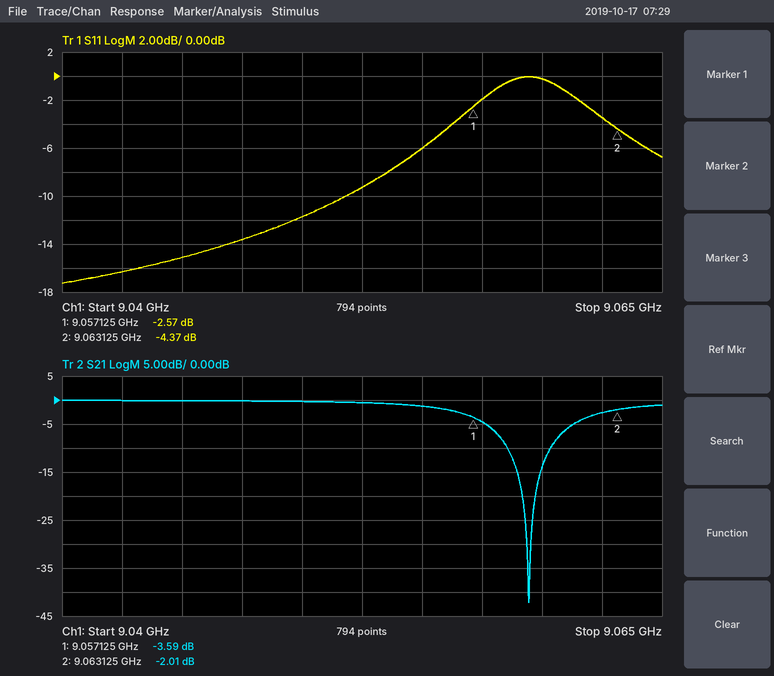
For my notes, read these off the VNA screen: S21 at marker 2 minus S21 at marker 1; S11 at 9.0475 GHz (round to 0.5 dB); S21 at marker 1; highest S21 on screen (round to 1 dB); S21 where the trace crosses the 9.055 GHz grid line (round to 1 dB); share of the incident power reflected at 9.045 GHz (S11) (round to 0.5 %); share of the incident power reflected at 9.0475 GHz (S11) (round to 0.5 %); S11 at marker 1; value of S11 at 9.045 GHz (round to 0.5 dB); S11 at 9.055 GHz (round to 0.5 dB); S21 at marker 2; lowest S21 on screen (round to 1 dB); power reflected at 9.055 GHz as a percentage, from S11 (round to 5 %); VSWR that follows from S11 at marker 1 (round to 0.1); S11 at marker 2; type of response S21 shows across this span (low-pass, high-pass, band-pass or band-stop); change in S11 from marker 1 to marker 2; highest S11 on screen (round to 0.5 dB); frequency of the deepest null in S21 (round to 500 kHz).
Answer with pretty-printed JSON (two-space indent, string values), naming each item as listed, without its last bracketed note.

{
  "S21 at marker 2 minus S21 at marker 1": "1.58 dB",
  "S11 at 9.0475 GHz": "-13.5 dB",
  "S21 at marker 1": "-3.59 dB",
  "highest S21 on screen": "0 dB",
  "S21 where the trace crosses the 9.055 GHz grid line": "-1 dB",
  "share of the incident power reflected at 9.045 GHz (S11)": "3.0 %",
  "share of the incident power reflected at 9.0475 GHz (S11)": "4.5 %",
  "S11 at marker 1": "-2.57 dB",
  "value of S11 at 9.045 GHz": "-15.0 dB",
  "S11 at 9.055 GHz": "-6.0 dB",
  "S21 at marker 2": "-2.01 dB",
  "lowest S21 on screen": "-42 dB",
  "power reflected at 9.055 GHz as a percentage, from S11": "25 %",
  "VSWR that follows from S11 at marker 1": "6.8",
  "S11 at marker 2": "-4.37 dB",
  "type of response S21 shows across this span": "band-stop",
  "change in S11 from marker 1 to marker 2": "-1.80 dB",
  "highest S11 on screen": "0.0 dB",
  "frequency of the deepest null in S21": "9.0595 GHz"
}
